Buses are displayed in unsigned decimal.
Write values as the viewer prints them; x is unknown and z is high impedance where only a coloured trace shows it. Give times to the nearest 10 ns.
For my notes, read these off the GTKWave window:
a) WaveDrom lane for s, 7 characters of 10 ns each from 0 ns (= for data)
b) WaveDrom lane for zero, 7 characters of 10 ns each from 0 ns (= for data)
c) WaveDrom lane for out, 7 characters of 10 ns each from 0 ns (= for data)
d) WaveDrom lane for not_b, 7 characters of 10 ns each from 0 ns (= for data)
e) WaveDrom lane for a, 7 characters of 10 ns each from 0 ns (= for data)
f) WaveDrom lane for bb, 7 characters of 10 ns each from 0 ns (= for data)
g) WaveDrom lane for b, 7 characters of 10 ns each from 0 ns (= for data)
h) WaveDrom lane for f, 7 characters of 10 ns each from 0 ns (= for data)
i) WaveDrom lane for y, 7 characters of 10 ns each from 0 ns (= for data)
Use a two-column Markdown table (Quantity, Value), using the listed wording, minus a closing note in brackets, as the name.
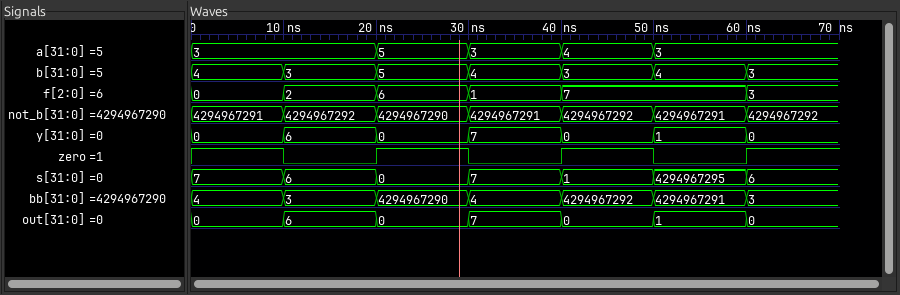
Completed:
| Quantity | Value |
|---|---|
| WaveDrom lane for s, 7 characters of 10 ns each from 0 ns | {name: 's', wave: '=======', data: '7 6 0 7 1 4294967295 6'} |
| WaveDrom lane for zero, 7 characters of 10 ns each from 0 ns | {name: 'zero', wave: '1010101'} |
| WaveDrom lane for out, 7 characters of 10 ns each from 0 ns | {name: 'out', wave: '=======', data: '0 6 0 7 0 1 0'} |
| WaveDrom lane for not_b, 7 characters of 10 ns each from 0 ns | {name: 'not_b', wave: '=======', data: '4294967291 4294967292 4294967290 4294967291 4294967292 4294967291 4294967292'} |
| WaveDrom lane for a, 7 characters of 10 ns each from 0 ns | {name: 'a', wave: '=.====.', data: '3 5 3 4 3'} |
| WaveDrom lane for bb, 7 characters of 10 ns each from 0 ns | {name: 'bb', wave: '=======', data: '4 3 4294967290 4 4294967292 4294967291 3'} |
| WaveDrom lane for b, 7 characters of 10 ns each from 0 ns | {name: 'b', wave: '=======', data: '4 3 5 4 3 4 3'} |
| WaveDrom lane for f, 7 characters of 10 ns each from 0 ns | {name: 'f', wave: '=====.=', data: '0 2 6 1 7 3'} |
| WaveDrom lane for y, 7 characters of 10 ns each from 0 ns | {name: 'y', wave: '=======', data: '0 6 0 7 0 1 0'} |
